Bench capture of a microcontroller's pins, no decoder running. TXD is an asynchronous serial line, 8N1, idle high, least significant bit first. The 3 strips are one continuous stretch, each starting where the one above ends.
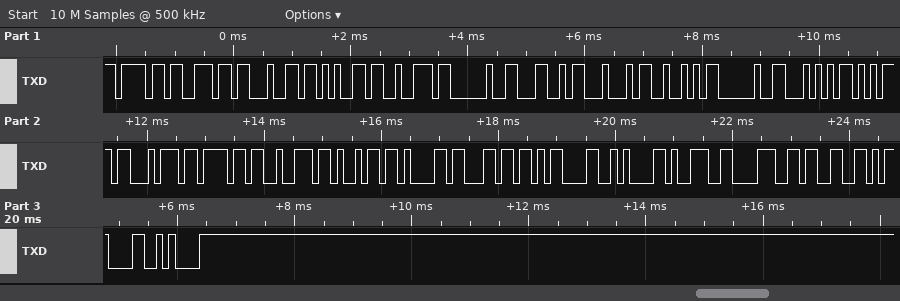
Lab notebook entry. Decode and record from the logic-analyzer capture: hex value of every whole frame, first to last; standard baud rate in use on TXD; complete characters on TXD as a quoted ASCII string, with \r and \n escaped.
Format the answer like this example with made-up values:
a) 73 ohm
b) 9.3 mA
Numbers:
a) 6F 6E 64 65 72 20 4C 44 52 20 54 75 74 6F 72 69 61 6C 0D 0A 39 38 33 0D 0A
b) 9600 baud
c) "onder LDR Tutorial\r\n983\r\n"
